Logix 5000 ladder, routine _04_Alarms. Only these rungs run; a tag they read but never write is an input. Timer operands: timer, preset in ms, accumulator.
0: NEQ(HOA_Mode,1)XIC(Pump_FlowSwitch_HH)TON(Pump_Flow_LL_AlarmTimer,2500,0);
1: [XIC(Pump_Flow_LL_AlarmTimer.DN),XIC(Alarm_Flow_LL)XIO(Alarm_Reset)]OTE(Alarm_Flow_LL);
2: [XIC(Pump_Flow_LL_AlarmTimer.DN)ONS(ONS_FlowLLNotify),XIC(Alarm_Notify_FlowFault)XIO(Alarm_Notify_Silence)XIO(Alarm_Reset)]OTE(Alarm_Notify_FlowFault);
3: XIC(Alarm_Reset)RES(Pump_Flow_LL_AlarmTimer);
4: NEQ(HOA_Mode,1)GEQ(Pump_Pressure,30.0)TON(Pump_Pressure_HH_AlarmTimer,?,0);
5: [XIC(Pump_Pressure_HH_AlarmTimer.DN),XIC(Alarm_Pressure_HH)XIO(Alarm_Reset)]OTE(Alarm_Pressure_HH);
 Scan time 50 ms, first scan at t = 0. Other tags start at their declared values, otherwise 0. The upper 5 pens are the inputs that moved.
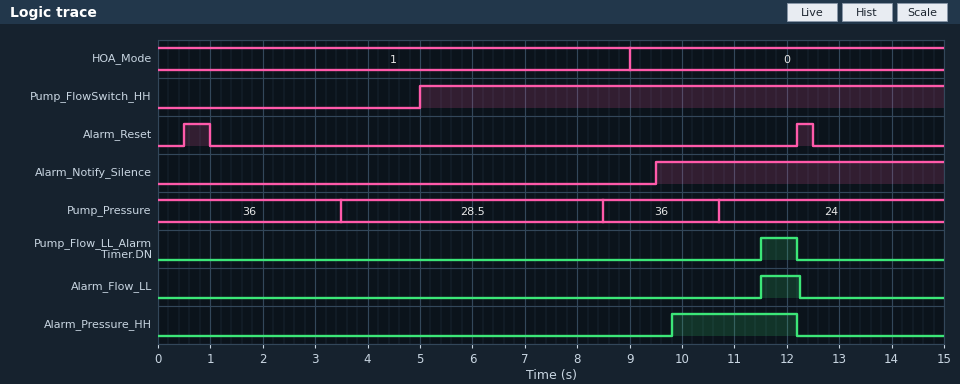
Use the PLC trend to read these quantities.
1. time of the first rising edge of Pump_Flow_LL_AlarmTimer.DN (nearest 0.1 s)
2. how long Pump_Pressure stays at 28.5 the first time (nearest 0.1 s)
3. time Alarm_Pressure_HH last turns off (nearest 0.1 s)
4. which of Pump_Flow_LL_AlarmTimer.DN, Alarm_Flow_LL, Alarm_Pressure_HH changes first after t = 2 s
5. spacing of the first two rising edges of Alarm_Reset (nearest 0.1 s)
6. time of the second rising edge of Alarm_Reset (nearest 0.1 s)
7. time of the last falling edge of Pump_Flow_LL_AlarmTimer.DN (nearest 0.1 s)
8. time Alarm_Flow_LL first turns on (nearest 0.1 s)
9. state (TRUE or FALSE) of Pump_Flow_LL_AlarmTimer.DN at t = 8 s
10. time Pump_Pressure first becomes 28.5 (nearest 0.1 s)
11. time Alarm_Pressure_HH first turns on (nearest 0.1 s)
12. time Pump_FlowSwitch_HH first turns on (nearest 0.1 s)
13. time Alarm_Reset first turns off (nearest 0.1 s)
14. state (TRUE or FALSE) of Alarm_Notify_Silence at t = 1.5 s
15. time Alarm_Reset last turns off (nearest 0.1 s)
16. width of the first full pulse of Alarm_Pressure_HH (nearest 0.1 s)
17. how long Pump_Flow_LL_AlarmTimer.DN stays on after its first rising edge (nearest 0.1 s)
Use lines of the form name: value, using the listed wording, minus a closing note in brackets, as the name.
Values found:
time of the first rising edge of Pump_Flow_LL_AlarmTimer.DN: 11.5 s
how long Pump_Pressure stays at 28.5 the first time: 5.0 s
time Alarm_Pressure_HH last turns off: 12.2 s
which of Pump_Flow_LL_AlarmTimer.DN, Alarm_Flow_LL, Alarm_Pressure_HH changes first after t = 2 s: Alarm_Pressure_HH
spacing of the first two rising edges of Alarm_Reset: 11.7 s
time of the second rising edge of Alarm_Reset: 12.2 s
time of the last falling edge of Pump_Flow_LL_AlarmTimer.DN: 12.2 s
time Alarm_Flow_LL first turns on: 11.5 s
state (TRUE or FALSE) of Pump_Flow_LL_AlarmTimer.DN at t = 8 s: FALSE
time Pump_Pressure first becomes 28.5: 3.5 s
time Alarm_Pressure_HH first turns on: 9.8 s
time Pump_FlowSwitch_HH first turns on: 5.0 s
time Alarm_Reset first turns off: 1.0 s
state (TRUE or FALSE) of Alarm_Notify_Silence at t = 1.5 s: FALSE
time Alarm_Reset last turns off: 12.5 s
width of the first full pulse of Alarm_Pressure_HH: 2.4 s
how long Pump_Flow_LL_AlarmTimer.DN stays on after its first rising edge: 0.7 s
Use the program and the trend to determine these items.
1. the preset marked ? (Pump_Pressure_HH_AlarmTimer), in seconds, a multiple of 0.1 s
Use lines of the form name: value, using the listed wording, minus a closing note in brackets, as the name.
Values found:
the preset marked ? (Pump_Pressure_HH_AlarmTimer), in seconds, a multiple of 0.1 s: 0.8 s
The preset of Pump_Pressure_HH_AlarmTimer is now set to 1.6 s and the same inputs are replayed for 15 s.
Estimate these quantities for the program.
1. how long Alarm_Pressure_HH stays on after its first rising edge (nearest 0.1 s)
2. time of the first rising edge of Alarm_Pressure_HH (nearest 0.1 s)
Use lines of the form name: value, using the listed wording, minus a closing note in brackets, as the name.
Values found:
how long Alarm_Pressure_HH stays on after its first rising edge: 1.6 s
time of the first rising edge of Alarm_Pressure_HH: 10.6 s
